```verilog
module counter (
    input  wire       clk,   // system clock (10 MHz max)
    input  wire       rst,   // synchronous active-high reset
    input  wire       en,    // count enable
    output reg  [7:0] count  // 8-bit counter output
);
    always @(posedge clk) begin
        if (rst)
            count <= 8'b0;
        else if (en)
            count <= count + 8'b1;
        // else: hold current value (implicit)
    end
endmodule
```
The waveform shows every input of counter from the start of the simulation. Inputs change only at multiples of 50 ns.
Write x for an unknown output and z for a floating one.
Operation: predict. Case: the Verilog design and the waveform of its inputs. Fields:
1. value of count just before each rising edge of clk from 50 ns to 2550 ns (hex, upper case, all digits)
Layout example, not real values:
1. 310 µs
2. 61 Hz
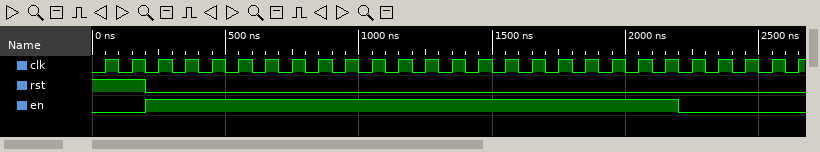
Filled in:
1. x, 00, 00, 01, 02, 03, 04, 05, 06, 07, 08, 09, 0A, 0B, 0C, 0D, 0E, 0F, 10, 11, 12, 13, 14, 14, 14, 14
